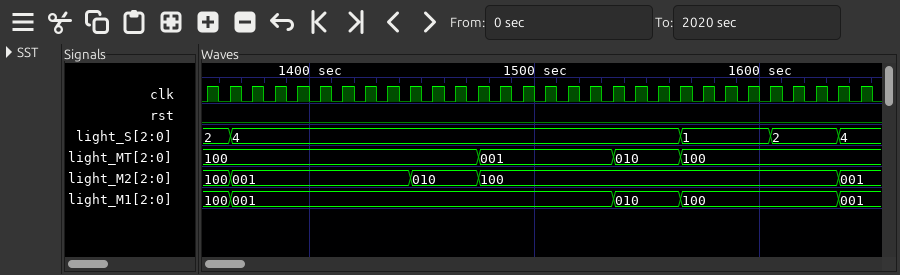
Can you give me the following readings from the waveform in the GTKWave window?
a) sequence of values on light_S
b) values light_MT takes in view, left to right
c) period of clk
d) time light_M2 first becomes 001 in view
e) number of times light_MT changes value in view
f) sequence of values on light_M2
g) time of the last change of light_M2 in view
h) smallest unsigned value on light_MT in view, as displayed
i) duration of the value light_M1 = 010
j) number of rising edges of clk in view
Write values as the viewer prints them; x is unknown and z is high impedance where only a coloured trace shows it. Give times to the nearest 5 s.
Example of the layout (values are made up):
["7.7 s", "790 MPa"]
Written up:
["2, 4, 1, 2, 4", "100, 001, 010, 100", "10 s", "1365 s", "3", "100, 001, 010, 100, 001", "1635 s", "001", "30 s", "30"]
